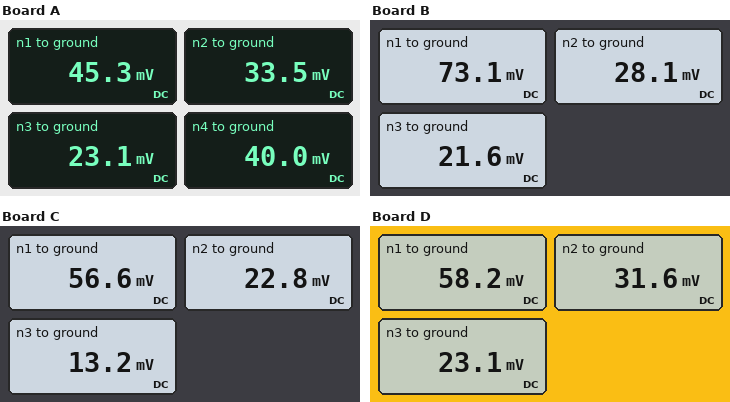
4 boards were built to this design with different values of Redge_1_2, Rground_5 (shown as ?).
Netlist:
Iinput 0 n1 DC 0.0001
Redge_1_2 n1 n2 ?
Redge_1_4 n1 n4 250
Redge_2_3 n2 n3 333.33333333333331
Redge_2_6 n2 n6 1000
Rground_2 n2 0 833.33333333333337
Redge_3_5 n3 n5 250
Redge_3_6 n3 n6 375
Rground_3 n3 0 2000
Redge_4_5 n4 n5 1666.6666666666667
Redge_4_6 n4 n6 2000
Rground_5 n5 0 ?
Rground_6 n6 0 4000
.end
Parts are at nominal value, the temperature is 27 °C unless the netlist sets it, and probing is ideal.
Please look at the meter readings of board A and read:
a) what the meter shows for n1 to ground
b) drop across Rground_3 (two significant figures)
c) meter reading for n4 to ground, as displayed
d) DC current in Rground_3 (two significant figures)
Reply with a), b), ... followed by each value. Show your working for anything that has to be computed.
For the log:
a) 45.3 mV
b) 23.1 mV = 23 mV
c) 40.0 mV
d) (23.1 mV) / 2 kΩ = 12 µA
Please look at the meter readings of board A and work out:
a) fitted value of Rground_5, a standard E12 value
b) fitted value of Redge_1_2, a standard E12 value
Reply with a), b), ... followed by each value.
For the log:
a) 390 Ω
b) 150 Ω
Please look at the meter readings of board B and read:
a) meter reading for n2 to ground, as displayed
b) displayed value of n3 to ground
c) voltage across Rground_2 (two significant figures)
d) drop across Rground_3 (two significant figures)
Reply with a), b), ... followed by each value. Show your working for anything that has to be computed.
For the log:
a) 28.1 mV
b) 21.6 mV
c) 28.1 mV = 28 mV
d) 21.6 mV = 22 mV
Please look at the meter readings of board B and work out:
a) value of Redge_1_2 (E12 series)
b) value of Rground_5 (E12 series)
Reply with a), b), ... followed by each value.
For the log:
a) 820 Ω
b) 330 Ω
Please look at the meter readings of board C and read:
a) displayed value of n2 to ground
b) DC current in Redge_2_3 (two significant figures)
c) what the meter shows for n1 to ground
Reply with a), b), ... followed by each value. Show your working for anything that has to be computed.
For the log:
a) 22.8 mV
b) (22.8 mV - 13.2 mV) / 333.3 Ω = 29 µA
c) 56.6 mV
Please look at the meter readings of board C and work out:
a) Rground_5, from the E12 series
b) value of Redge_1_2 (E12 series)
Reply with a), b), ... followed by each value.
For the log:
a) 68 Ω
b) 560 Ω
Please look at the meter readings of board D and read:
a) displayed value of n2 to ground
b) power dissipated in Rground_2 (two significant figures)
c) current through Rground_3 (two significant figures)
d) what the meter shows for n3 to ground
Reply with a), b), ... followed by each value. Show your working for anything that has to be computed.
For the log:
a) 31.6 mV
b) (31.6 mV)^2 / 833.3 Ω = 1.2 µW
c) (23.1 mV) / 2 kΩ = 12 µA
d) 23.1 mV
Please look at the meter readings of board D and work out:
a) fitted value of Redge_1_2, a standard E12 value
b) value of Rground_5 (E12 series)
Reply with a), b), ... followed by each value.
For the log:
a) 390 Ω
b) 390 Ω
